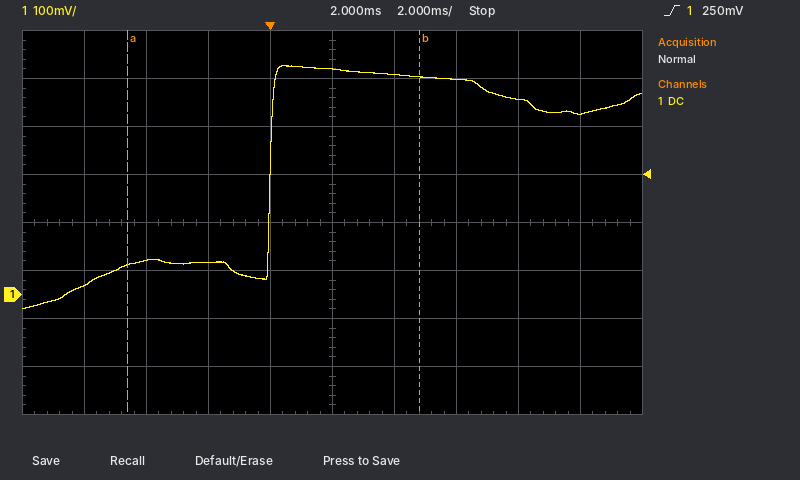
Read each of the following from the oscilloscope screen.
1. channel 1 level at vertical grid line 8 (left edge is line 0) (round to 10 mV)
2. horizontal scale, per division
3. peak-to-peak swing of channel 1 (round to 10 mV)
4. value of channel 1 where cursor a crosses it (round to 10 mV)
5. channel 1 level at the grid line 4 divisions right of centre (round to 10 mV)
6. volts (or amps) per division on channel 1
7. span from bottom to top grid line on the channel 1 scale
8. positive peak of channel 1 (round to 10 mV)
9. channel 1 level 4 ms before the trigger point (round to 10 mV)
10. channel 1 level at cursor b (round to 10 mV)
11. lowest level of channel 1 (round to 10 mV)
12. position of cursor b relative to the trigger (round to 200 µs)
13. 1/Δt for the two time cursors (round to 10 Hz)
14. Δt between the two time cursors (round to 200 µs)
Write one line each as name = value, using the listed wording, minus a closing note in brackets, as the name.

channel 1 level at vertical grid line 8 (left edge is line 0) = 410 mV
horizontal scale, per division = 2 ms
peak-to-peak swing of channel 1 = 510 mV
value of channel 1 where cursor a crosses it = 60 mV
channel 1 level at the grid line 4 divisions right of centre = 380 mV
volts (or amps) per division on channel 1 = 100 mV
span from bottom to top grid line on the channel 1 scale = 800 mV
positive peak of channel 1 = 480 mV
channel 1 level 4 ms before the trigger point = 70 mV
channel 1 level at cursor b = 450 mV
lowest level of channel 1 = -30 mV
position of cursor b relative to the trigger = +4.8 ms
1/Δt for the two time cursors = 110 Hz
Δt between the two time cursors = 9.4 ms
